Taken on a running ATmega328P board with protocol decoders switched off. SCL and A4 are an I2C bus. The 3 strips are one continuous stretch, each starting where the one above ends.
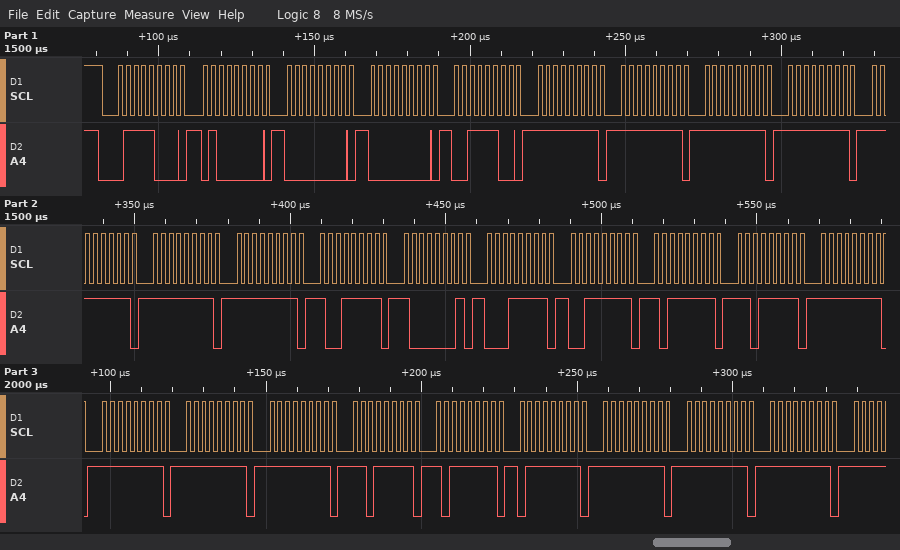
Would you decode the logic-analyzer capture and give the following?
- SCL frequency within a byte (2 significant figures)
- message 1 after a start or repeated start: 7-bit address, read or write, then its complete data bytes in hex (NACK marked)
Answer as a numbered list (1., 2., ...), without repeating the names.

1. 400 kHz
2. 0x3C write: 40 00 00 3C FF FF FF FF FF FF FF 9F 81 1F 3F BF DF FF FF FF FF DF BF 7F FF FF FF
